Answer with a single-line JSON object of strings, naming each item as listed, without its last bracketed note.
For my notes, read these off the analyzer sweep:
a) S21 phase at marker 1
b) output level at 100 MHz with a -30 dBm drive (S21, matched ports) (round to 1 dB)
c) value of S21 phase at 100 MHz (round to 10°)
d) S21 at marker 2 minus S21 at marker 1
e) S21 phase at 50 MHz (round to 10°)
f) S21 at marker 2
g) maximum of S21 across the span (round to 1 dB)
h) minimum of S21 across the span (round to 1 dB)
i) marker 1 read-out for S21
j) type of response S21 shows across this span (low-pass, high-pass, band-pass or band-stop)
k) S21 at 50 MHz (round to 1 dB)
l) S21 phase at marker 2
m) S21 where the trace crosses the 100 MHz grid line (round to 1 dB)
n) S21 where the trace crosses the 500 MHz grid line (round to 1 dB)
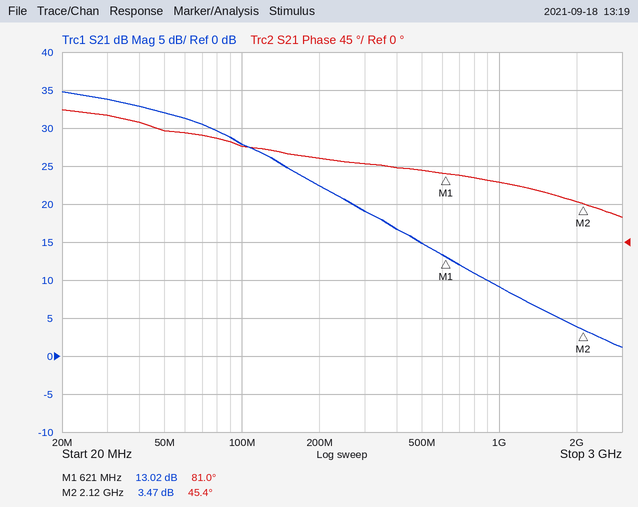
{"S21 phase at marker 1": "81.0°", "output level at 100 MHz with a -30 dBm drive (S21, matched ports)": "-2 dBm", "value of S21 phase at 100 MHz": "110°", "S21 at marker 2 minus S21 at marker 1": "-9.55 dB", "S21 phase at 50 MHz": "130°", "S21 at marker 2": "3.47 dB", "maximum of S21 across the span": "35 dB", "minimum of S21 across the span": "1 dB", "marker 1 read-out for S21": "13.02 dB", "type of response S21 shows across this span": "low-pass", "S21 at 50 MHz": "32 dB", "S21 phase at marker 2": "45.4°", "S21 where the trace crosses the 100 MHz grid line": "28 dB", "S21 where the trace crosses the 500 MHz grid line": "15 dB"}
